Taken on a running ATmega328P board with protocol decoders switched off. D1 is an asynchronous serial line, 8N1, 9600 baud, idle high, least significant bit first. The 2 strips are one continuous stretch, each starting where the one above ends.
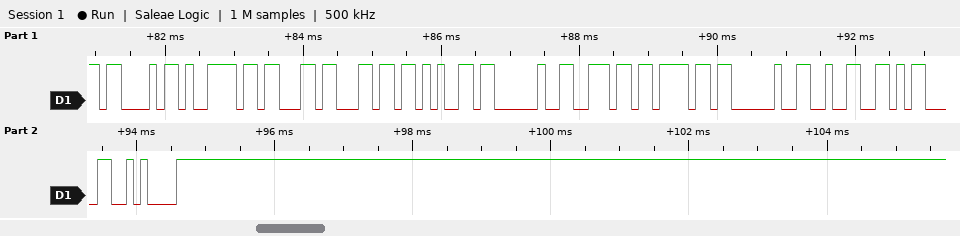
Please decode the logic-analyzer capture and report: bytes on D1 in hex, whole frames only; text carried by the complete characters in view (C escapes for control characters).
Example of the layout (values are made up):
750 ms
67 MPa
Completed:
43 79 63 6C 65 20 6E 6F 20 32 0D 0A
"Cycle no 2\r\n"
